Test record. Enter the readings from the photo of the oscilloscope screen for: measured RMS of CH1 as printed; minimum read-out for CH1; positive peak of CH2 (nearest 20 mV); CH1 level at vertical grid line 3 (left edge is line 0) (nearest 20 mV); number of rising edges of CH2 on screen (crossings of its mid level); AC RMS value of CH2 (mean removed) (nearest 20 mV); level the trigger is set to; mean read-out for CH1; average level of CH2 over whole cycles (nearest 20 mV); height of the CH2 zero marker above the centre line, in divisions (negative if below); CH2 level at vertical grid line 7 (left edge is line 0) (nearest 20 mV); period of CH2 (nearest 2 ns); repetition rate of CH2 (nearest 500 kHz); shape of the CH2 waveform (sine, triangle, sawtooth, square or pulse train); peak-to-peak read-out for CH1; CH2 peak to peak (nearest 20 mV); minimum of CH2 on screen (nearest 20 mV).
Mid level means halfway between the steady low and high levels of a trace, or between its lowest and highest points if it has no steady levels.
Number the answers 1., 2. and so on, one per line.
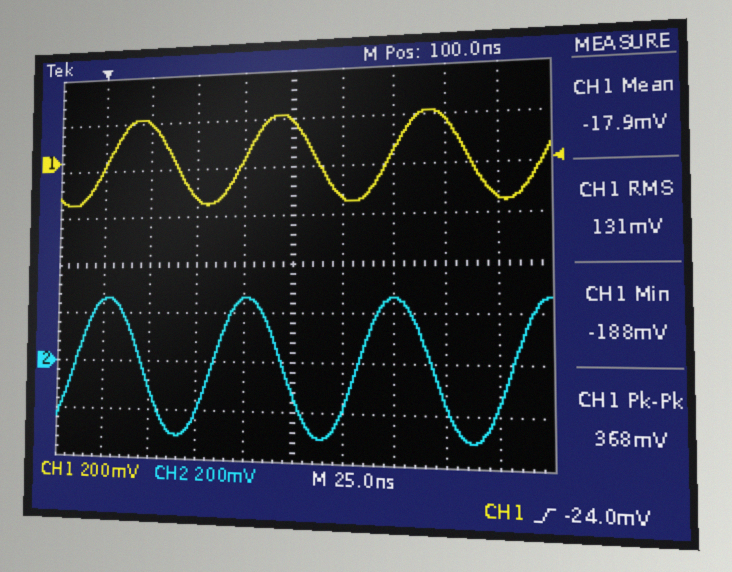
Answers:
1. 131 mV
2. -188 mV
3. 260 mV
4. -160 mV
5. 4
6. 200 mV
7. -24.0 mV
8. -17.9 mV
9. -20 mV
10. -2.0 div
11. 260 mV
12. 74 ns
13. 13.5 MHz
14. sine
15. 368 mV
16. 560 mV
17. -300 mV
